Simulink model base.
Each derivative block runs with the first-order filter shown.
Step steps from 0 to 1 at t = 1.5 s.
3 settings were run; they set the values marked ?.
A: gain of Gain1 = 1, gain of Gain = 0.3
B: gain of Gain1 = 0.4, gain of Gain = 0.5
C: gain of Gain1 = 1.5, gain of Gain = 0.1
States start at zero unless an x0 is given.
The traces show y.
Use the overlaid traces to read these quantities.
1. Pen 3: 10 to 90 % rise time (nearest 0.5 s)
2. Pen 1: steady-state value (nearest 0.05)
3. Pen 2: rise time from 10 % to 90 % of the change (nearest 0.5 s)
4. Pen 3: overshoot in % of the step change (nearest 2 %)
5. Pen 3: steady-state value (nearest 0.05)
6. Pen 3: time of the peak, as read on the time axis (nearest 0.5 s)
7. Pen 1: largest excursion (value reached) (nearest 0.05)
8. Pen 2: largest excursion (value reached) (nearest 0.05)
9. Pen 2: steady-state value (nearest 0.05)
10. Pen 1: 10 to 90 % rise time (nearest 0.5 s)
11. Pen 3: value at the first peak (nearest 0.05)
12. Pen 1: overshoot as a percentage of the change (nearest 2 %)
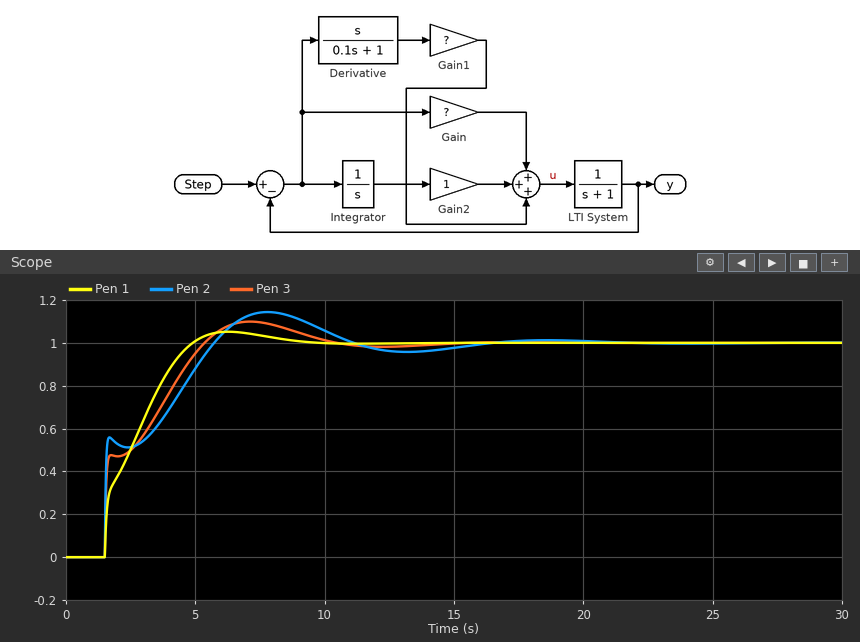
3.0 s
1.00
3.5 s
10 %
1.00
7.0 s
1.05
1.15
1.00
2.5 s
1.10
6 %
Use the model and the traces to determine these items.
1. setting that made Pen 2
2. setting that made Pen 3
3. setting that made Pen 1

C
A
B
